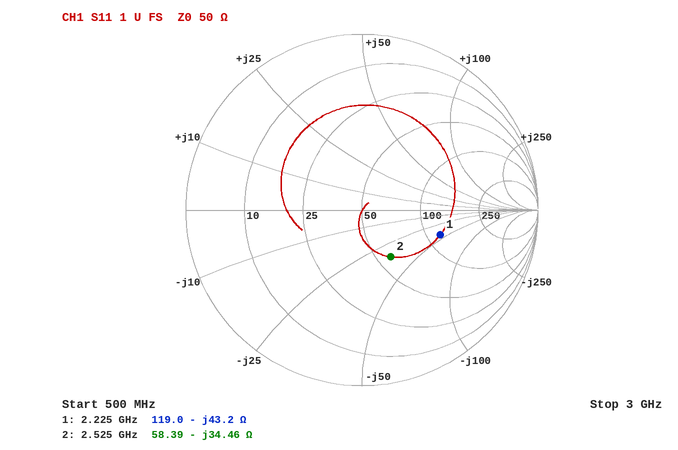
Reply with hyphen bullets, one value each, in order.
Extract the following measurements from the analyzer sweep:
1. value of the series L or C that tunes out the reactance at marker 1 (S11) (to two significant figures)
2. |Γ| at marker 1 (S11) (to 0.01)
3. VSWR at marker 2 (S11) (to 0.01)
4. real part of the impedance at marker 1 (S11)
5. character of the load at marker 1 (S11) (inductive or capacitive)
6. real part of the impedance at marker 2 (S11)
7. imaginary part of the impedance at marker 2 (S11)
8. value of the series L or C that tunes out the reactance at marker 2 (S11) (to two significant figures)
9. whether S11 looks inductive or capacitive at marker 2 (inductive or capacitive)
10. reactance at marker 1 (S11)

- 3.1 nH
- 0.47
- 1.91
- 119.0 Ω
- capacitive
- 58.39 Ω
- -34.46 Ω
- 2.2 nH
- capacitive
- -43.2 Ω
